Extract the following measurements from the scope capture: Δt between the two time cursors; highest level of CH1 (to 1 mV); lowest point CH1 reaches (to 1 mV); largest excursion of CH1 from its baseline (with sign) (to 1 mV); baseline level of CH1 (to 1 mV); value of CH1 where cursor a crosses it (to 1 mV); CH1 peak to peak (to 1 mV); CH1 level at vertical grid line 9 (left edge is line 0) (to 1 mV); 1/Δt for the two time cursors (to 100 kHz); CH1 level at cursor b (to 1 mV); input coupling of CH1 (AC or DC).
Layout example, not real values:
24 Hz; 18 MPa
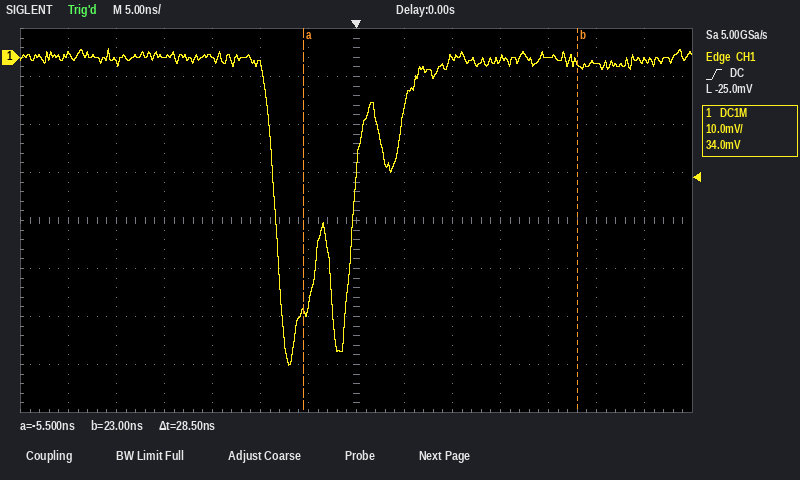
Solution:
28.5 ns; 2 mV; -64 mV; -64 mV; 0 mV; -53 mV; 66 mV; 0 mV; 35.1 MHz; -1 mV; DC
